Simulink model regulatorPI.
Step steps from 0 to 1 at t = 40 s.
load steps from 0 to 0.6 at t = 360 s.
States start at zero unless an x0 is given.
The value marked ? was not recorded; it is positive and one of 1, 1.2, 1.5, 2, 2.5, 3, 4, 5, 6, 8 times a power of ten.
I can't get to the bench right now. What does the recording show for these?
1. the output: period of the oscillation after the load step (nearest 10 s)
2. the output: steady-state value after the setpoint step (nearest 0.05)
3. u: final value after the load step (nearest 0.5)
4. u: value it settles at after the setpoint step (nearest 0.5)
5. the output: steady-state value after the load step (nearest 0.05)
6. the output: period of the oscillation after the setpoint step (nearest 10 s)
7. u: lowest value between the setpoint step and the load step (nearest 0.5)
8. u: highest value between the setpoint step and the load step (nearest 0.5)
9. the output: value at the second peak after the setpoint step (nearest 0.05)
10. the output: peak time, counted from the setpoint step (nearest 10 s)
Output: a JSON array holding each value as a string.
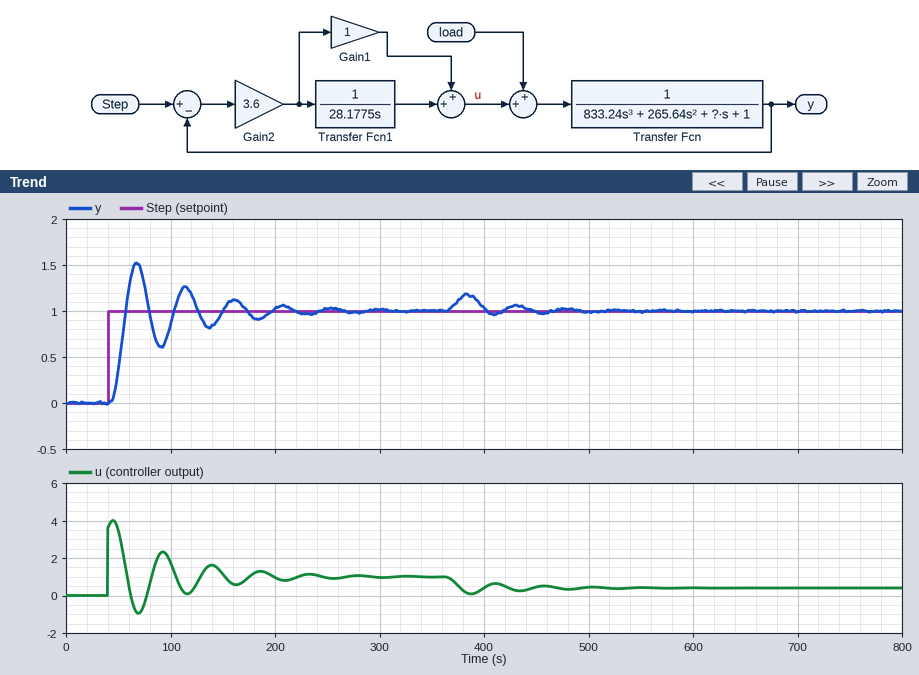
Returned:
["50 s", "1.00", "0.5", "1.0", "1.00", "50 s", "-1.0", "4.0", "1.25", "30 s"]
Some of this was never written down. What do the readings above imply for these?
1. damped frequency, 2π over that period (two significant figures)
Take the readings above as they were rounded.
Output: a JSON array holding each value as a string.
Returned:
["0.13 rad/s"]
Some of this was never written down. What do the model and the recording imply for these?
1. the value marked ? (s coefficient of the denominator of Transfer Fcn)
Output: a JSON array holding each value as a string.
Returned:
["30"]
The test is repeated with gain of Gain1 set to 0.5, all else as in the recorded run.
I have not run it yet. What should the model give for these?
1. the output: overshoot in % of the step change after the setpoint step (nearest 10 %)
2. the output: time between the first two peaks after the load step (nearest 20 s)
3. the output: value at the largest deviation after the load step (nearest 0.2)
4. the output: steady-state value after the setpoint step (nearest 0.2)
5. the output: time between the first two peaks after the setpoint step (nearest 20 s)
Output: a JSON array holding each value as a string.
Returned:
["50 %", "60 s", "1.2", "1.0", "60 s"]
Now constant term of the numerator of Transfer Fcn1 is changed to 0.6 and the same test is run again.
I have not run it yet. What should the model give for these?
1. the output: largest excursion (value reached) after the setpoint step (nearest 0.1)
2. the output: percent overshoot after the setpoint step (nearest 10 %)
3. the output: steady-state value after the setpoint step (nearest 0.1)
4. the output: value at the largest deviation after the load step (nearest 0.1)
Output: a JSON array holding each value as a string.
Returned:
["1.4", "40 %", "1.0", "1.2"]
